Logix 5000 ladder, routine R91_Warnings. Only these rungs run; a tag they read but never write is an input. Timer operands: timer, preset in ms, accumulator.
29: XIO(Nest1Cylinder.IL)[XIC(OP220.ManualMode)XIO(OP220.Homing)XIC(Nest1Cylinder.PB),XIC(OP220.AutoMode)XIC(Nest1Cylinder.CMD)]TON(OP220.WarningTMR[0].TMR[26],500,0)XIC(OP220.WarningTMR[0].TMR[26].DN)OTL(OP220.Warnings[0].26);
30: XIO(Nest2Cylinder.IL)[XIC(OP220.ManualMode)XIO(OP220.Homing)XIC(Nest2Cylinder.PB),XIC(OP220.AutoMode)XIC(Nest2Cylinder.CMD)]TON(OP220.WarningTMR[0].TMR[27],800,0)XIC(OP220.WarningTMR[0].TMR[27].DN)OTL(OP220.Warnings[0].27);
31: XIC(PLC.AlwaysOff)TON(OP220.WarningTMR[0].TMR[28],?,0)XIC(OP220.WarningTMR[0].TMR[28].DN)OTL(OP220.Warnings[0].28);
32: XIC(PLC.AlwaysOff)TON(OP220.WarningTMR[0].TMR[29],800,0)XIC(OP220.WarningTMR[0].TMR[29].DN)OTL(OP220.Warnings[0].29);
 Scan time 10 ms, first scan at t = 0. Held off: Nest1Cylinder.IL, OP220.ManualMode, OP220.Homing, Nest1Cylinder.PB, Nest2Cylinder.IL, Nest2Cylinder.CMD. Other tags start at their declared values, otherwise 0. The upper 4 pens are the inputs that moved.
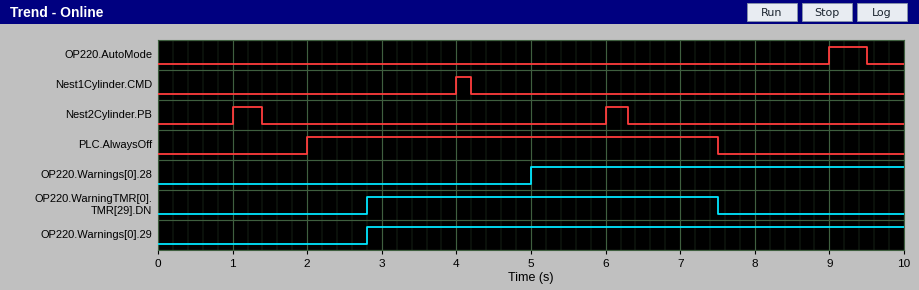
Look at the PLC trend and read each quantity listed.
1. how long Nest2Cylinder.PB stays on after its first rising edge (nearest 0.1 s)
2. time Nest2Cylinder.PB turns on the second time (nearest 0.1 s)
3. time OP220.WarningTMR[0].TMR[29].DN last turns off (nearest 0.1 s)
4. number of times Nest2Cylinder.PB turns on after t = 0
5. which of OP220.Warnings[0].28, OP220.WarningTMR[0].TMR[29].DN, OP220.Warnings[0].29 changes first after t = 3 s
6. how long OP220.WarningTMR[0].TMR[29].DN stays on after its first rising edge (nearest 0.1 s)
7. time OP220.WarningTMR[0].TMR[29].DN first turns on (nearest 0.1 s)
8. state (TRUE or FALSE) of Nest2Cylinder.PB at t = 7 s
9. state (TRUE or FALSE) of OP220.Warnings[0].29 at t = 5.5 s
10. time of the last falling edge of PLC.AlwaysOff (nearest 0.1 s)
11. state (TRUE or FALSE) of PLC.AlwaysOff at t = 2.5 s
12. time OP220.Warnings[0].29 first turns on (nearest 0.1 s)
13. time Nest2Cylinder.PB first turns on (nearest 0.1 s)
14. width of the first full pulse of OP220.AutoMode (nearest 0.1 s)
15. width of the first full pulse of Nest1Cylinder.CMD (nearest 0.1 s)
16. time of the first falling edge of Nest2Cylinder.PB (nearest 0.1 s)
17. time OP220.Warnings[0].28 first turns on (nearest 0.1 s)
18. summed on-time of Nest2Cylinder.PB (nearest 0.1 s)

0.4 s
6.0 s
7.5 s
2
OP220.Warnings[0].28
4.7 s
2.8 s
FALSE
TRUE
7.5 s
TRUE
2.8 s
1.0 s
0.5 s
0.2 s
1.4 s
5.0 s
0.7 s
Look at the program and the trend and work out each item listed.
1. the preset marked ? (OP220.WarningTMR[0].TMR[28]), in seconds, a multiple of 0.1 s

3.0 s
